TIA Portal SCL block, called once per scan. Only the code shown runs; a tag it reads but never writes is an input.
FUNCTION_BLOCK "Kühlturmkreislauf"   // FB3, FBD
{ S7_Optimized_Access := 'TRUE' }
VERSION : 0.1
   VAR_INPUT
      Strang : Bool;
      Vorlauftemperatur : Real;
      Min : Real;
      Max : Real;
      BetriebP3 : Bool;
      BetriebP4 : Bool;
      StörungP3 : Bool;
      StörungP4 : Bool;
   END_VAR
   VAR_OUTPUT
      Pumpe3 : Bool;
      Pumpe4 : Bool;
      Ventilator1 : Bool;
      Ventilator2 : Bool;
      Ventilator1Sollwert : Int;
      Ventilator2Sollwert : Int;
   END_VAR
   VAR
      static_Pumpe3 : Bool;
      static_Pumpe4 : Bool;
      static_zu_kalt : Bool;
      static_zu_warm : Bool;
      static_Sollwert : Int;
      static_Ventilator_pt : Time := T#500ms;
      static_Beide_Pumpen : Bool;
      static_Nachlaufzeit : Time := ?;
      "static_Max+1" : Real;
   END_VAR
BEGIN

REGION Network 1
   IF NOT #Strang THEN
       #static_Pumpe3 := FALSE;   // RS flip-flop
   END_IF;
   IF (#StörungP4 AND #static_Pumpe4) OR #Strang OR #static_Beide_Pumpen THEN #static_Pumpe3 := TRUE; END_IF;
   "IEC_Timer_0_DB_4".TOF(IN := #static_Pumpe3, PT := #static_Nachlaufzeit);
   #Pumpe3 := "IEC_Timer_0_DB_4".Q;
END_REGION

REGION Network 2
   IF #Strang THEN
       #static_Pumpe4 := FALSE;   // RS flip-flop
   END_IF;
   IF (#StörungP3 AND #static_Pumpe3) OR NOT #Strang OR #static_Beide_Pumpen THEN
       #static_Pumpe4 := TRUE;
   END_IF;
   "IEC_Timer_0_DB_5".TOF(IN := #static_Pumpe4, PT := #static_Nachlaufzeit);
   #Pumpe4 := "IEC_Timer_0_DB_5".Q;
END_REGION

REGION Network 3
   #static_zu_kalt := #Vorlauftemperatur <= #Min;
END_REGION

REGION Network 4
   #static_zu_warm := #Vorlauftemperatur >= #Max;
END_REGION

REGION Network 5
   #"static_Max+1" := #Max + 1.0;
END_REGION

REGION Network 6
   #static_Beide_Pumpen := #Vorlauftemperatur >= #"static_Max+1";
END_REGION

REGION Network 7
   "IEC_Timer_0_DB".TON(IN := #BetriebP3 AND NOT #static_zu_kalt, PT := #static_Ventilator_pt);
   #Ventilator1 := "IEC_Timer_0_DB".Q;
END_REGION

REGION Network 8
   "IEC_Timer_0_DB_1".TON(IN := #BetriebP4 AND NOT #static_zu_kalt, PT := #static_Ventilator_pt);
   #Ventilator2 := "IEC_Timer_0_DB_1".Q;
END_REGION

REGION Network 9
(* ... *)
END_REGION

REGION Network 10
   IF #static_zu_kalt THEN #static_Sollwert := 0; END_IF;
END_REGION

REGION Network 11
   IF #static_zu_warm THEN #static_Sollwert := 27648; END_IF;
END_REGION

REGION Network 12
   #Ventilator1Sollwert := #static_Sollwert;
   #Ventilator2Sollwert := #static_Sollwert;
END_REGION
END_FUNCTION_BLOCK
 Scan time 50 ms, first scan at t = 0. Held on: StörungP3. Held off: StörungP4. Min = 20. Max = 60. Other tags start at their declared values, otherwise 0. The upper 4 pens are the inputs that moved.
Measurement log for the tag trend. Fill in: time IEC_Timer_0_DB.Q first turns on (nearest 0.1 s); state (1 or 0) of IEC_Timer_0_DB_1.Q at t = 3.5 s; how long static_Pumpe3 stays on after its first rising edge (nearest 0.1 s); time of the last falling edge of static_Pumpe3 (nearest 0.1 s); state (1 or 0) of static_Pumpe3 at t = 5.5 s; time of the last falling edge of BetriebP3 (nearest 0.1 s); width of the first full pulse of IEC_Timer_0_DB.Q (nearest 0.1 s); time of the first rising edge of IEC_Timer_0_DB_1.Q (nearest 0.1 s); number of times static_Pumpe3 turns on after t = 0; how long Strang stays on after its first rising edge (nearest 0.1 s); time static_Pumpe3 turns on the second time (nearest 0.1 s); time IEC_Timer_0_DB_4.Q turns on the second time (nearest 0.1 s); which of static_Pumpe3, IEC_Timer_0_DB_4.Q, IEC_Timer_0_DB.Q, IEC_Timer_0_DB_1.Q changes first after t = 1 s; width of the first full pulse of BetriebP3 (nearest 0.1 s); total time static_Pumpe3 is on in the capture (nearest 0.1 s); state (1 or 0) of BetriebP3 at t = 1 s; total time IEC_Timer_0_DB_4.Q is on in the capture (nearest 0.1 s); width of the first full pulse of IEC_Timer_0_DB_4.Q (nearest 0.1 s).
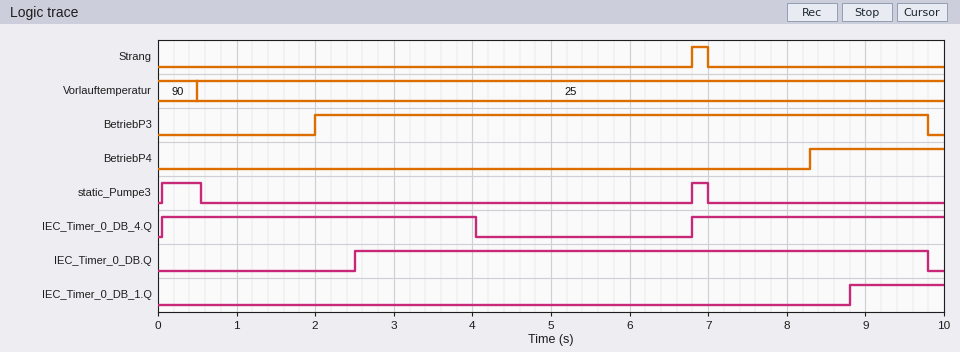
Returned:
2.5 s
0
0.5 s
7.0 s
0
9.8 s
7.3 s
8.8 s
2
0.2 s
6.8 s
6.8 s
IEC_Timer_0_DB.Q
7.8 s
0.7 s
0
7.2 s
4.0 s
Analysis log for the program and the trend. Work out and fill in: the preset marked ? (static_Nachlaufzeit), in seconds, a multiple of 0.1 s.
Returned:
3.5 s
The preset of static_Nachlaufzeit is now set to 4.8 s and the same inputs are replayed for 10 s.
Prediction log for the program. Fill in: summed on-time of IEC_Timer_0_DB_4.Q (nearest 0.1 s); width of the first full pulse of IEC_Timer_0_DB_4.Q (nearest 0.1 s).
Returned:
8.5 s
5.3 s
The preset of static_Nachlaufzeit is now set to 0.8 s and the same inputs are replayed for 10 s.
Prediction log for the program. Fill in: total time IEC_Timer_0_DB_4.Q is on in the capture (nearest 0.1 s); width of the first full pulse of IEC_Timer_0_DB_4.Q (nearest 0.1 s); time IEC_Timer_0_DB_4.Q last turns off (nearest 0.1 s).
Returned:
2.3 s
1.3 s
7.8 s
